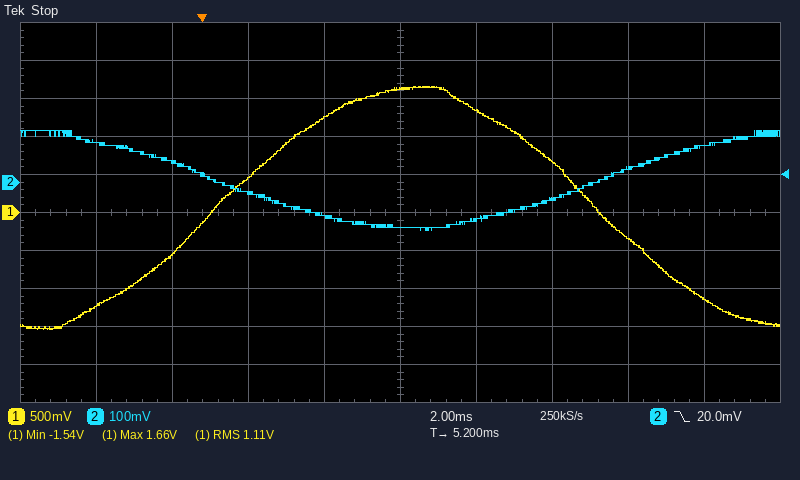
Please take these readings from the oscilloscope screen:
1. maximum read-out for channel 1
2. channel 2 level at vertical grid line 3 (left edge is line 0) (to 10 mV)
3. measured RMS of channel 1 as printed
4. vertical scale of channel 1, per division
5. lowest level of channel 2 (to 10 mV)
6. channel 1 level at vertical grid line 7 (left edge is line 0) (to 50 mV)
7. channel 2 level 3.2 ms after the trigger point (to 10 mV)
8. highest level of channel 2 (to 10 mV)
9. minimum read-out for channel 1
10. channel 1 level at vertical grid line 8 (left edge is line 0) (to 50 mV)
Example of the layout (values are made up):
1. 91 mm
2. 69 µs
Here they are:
1. 1.66 V
2. -30 mV
3. 1.11 V
4. 500 mV
5. -130 mV
6. 650 mV
7. -90 mV
8. 140 mV
9. -1.54 V
10. -350 mV
